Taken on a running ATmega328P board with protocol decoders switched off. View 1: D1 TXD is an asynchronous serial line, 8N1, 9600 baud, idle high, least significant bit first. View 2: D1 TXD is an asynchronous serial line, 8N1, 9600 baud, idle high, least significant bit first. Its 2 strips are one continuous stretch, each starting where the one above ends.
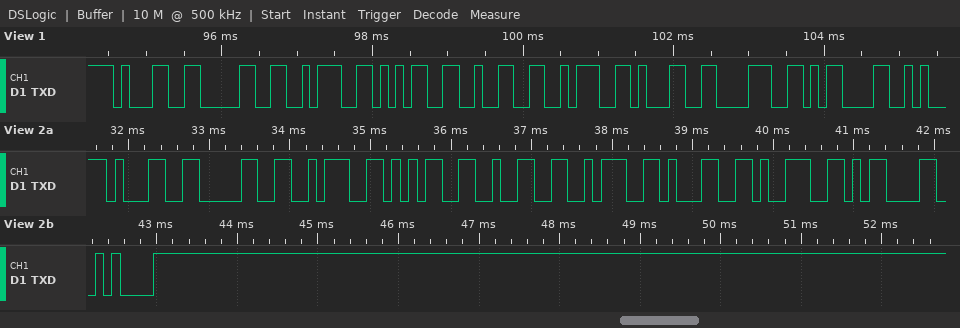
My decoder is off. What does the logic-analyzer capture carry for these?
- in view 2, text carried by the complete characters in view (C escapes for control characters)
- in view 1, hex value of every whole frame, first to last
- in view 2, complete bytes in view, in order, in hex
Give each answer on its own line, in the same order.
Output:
"10:52:19\r\n"
0x31 0x30 0x3A 0x35 0x32 0x3A 0x31 0x38 0x0D
0x31 0x30 0x3A 0x35 0x32 0x3A 0x31 0x39 0x0D 0x0A
